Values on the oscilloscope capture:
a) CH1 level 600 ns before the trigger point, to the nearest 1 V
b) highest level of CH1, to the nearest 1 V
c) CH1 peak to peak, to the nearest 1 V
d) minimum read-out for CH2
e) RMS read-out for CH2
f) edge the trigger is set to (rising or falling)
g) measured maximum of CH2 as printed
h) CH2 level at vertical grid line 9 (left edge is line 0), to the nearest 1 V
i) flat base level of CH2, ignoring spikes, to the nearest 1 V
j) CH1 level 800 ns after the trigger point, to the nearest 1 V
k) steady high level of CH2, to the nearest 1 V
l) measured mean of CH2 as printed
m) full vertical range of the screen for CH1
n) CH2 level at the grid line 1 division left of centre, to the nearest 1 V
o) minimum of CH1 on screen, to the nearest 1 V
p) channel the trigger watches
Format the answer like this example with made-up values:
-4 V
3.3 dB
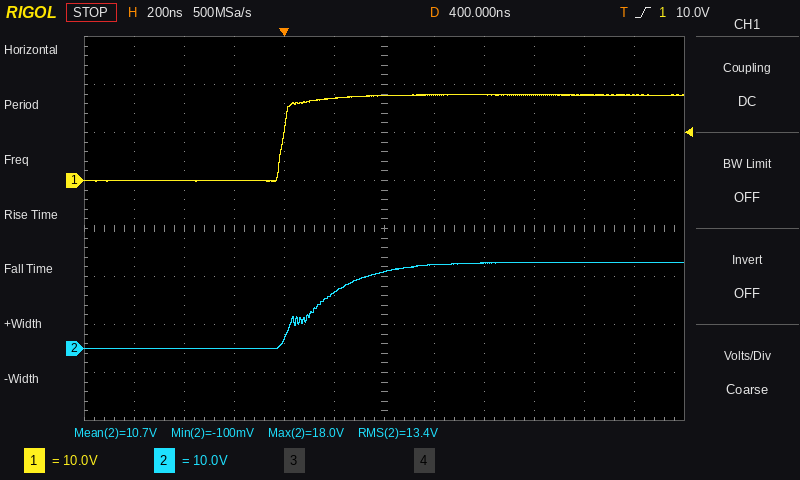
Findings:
0 V
18 V
18 V
-100 mV
13.4 V
rising
18.0 V
18 V
0 V
18 V
18 V
10.7 V
80 V
12 V
0 V
CH1
